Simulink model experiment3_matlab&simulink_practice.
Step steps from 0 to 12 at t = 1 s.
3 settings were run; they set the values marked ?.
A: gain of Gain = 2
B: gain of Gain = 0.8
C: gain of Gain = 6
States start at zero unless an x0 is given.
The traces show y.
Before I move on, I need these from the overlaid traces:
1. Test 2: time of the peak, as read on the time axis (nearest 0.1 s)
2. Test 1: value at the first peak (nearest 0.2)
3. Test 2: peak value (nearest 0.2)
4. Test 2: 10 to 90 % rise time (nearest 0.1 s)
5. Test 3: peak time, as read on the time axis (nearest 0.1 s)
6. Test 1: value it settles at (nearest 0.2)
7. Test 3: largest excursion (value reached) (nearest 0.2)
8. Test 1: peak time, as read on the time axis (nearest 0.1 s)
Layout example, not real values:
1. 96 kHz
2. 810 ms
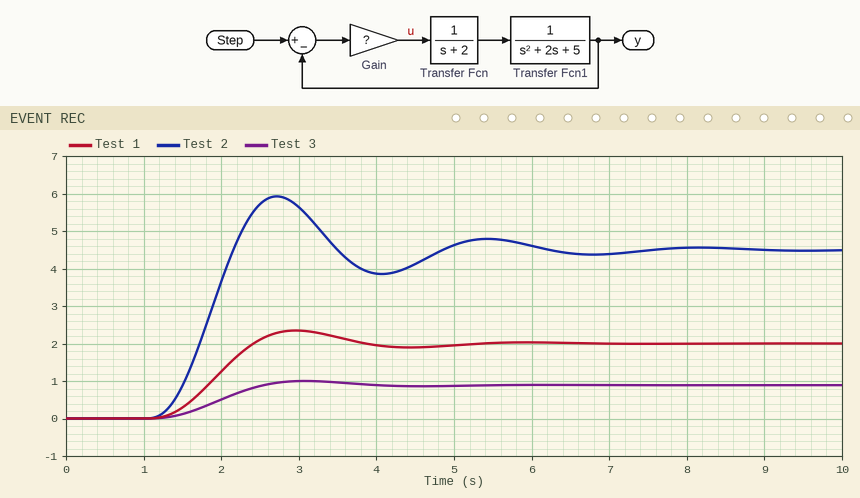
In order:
1. 2.7 s
2. 2.4
3. 6.0
4. 0.7 s
5. 3.1 s
6. 2.0
7. 1.0
8. 3.0 s
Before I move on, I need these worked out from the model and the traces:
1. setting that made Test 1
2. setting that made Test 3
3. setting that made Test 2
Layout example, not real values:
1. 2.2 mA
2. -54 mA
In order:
1. A
2. B
3. C
